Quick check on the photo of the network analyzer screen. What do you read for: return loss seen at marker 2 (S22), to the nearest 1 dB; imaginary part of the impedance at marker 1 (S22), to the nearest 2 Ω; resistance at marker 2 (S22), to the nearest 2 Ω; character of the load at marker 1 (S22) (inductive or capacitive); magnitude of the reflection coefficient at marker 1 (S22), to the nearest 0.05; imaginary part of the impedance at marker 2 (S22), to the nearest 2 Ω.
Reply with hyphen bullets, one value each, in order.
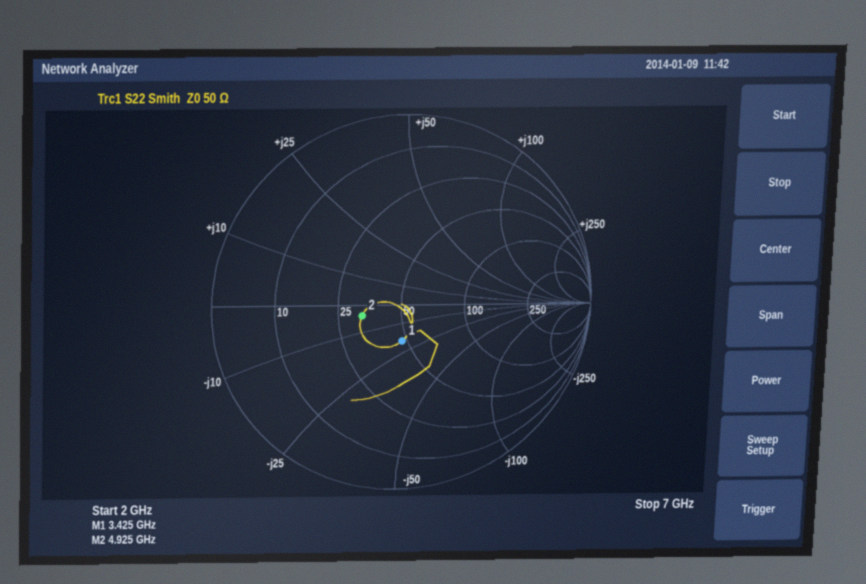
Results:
- 13 dB
- -20 Ω
- 32 Ω
- capacitive
- 0.20
- -4 Ω
